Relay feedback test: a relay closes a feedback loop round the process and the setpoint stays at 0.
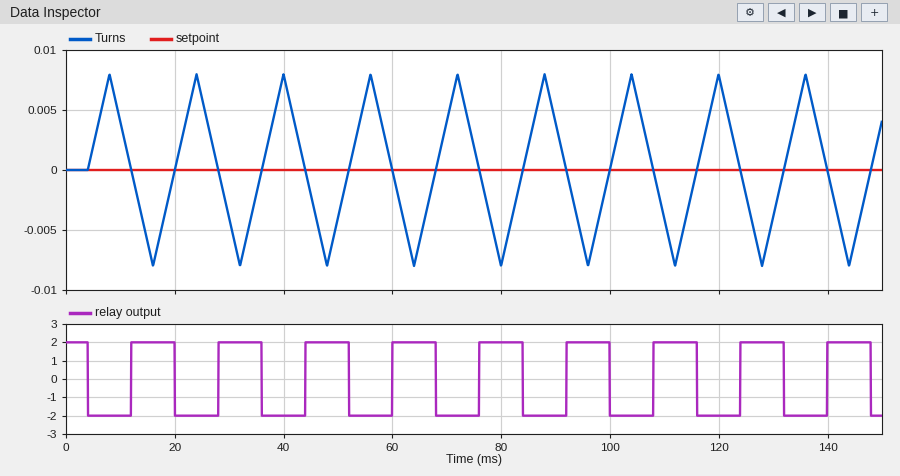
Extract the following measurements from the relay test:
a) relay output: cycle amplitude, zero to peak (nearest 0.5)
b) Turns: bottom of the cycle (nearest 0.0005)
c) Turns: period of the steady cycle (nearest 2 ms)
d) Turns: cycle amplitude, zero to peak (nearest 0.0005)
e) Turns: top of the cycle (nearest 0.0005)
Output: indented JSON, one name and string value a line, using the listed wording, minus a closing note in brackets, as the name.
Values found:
{
  "relay output: cycle amplitude, zero to peak": "2.0",
  "Turns: bottom of the cycle": "-0.0080",
  "Turns: period of the steady cycle": "16 ms",
  "Turns: cycle amplitude, zero to peak": "0.0080",
  "Turns: top of the cycle": "0.0080"
}
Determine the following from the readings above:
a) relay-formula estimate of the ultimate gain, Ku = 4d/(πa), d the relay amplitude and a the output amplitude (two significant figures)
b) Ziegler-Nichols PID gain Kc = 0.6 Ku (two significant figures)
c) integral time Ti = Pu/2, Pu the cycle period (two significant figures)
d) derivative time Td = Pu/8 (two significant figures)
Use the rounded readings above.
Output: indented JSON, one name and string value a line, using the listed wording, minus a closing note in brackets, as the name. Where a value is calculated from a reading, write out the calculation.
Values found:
{
  "relay-formula estimate of the ultimate gain, Ku = 4d/(πa), d the relay amplitude and a the output amplitude": "4 × 2 / (π × 0.008) = 320",
  "Ziegler-Nichols PID gain Kc = 0.6 Ku": "0.6 × 320 = 190",
  "integral time Ti = Pu/2, Pu the cycle period": "16 / 2 = 8.0 ms",
  "derivative time Td = Pu/8": "16 / 8 = 2.0 ms"
}
